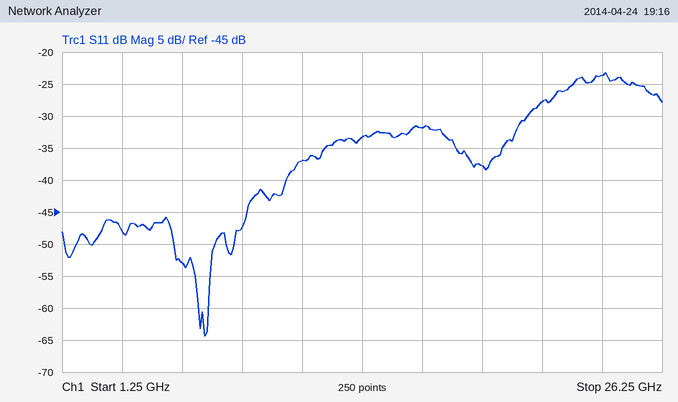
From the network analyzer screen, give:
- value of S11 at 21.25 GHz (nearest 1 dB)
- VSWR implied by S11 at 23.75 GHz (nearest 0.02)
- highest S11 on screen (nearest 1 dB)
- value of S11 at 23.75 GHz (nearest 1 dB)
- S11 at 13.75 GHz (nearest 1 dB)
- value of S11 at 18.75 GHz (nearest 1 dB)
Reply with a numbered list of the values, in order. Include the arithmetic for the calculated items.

1. -28 dB
2. |Γ| = 10^(-24/20) = 0.0631; VSWR = (1 + 0.0631)/(1 − 0.0631) ≈ 1.13, so 1.14 to the nearest 0.02
3. -23 dB
4. -24 dB
5. -33 dB
6. -38 dB
